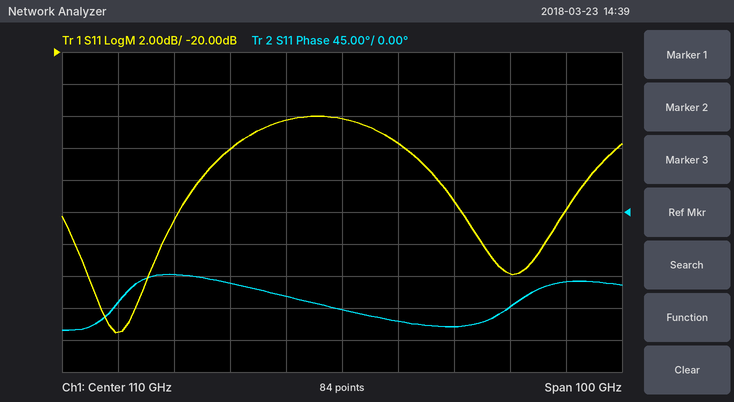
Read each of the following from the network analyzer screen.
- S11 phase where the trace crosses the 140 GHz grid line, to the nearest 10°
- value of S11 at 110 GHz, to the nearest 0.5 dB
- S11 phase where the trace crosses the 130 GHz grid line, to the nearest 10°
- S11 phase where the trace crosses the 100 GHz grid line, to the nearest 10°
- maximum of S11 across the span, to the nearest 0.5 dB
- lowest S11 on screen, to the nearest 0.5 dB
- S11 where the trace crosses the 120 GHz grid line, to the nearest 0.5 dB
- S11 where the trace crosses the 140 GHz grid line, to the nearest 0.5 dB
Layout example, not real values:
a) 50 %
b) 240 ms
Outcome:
a) -130°
b) -24.0 dB
c) -160°
d) -120°
e) -24.0 dB
f) -37.5 dB
g) -25.5 dB
h) -34.0 dB
